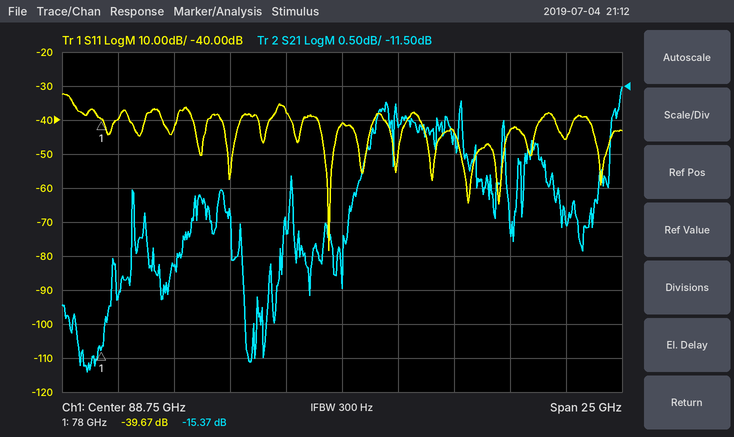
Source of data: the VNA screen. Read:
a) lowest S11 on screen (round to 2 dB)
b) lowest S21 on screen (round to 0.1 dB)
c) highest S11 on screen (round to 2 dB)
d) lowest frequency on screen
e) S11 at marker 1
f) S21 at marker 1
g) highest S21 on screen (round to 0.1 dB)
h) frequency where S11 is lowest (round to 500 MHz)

-78 dB
-15.7 dB
-32 dB
76.25 GHz
-39.67 dB
-15.37 dB
-11.5 dB
88.0 GHz
